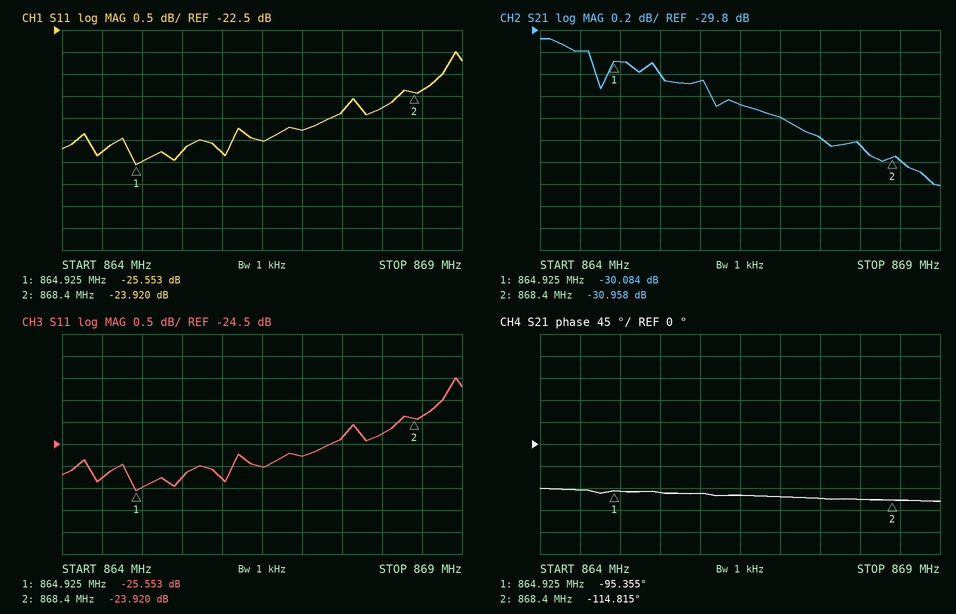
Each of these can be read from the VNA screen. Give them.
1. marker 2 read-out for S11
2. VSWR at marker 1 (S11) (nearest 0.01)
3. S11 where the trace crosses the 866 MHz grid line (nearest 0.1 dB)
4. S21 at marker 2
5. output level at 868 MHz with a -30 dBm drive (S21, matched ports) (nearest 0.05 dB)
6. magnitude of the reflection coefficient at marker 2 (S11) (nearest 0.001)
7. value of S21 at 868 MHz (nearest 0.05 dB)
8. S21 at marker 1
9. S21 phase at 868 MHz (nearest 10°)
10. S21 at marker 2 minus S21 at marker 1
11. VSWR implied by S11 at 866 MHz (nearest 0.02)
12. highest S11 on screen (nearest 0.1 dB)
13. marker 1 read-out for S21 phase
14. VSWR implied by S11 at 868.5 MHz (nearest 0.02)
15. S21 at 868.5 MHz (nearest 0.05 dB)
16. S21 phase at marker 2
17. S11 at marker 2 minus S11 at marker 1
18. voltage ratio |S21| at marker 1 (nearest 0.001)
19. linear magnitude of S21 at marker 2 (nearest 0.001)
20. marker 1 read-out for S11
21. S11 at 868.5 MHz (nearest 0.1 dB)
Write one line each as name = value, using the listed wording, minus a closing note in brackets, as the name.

marker 2 read-out for S11 = -23.920 dB
VSWR at marker 1 (S11) = 1.11
S11 where the trace crosses the 866 MHz grid line = -25.3 dB
S21 at marker 2 = -30.958 dB
output level at 868 MHz with a -30 dBm drive (S21, matched ports) = -60.85 dBm
magnitude of the reflection coefficient at marker 2 (S11) = 0.064
value of S21 at 868 MHz = -30.85 dB
S21 at marker 1 = -30.084 dB
S21 phase at 868 MHz = -110°
S21 at marker 2 minus S21 at marker 1 = -0.874 dB
VSWR implied by S11 at 866 MHz = 1.12
highest S11 on screen = -23.0 dB
marker 1 read-out for S21 phase = -95.355°
VSWR implied by S11 at 868.5 MHz = 1.14
S21 at 868.5 MHz = -31.00 dB
S21 phase at marker 2 = -114.815°
S11 at marker 2 minus S11 at marker 1 = 1.633 dB
voltage ratio |S21| at marker 1 = 0.031
linear magnitude of S21 at marker 2 = 0.028
marker 1 read-out for S11 = -25.553 dB
S11 at 868.5 MHz = -23.9 dB
